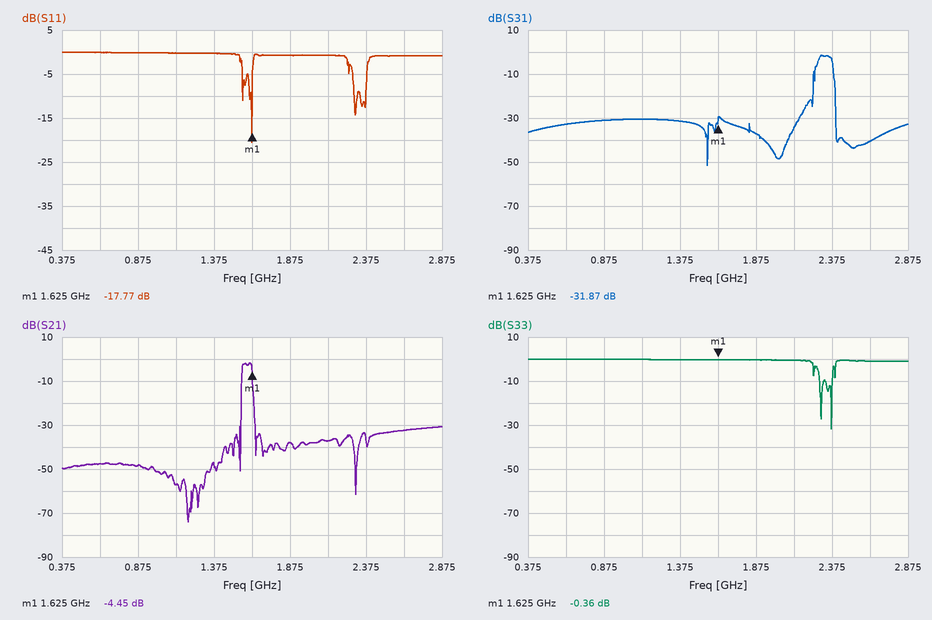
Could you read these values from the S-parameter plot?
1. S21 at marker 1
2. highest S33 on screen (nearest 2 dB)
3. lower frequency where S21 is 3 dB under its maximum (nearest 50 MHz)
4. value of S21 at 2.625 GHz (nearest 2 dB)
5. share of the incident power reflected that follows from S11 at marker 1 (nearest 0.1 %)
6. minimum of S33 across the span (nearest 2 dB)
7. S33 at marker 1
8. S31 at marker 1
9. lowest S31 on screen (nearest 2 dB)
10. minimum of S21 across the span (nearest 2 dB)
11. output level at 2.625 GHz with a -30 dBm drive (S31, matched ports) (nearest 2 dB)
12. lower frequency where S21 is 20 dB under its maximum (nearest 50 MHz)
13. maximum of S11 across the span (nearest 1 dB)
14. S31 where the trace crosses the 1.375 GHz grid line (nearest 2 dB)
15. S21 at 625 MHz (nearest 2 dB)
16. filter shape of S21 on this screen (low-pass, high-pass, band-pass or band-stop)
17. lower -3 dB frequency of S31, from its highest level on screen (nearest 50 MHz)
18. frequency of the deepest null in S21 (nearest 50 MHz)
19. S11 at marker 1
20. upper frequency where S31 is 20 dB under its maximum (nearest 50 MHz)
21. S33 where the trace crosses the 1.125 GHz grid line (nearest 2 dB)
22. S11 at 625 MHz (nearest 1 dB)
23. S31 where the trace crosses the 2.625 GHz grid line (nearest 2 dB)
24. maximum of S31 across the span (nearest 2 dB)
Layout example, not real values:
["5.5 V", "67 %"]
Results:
["-4.45 dB", "0 dB", "1.55 GHz", "-32 dB", "1.7 %", "-32 dB", "-0.36 dB", "-31.87 dB", "-52 dB", "-74 dB", "-70 dBm", "1.55 GHz", "0 dB", "-32 dB", "-48 dB", "band-pass", "2.30 GHz", "1.20 GHz", "-17.77 dB", "2.40 GHz", "0 dB", "0 dB", "-40 dB", "-2 dB"]
